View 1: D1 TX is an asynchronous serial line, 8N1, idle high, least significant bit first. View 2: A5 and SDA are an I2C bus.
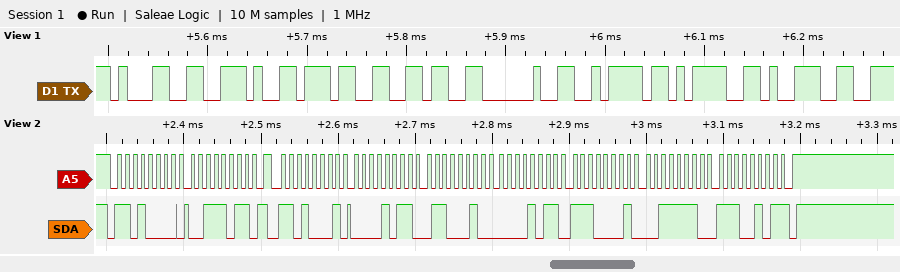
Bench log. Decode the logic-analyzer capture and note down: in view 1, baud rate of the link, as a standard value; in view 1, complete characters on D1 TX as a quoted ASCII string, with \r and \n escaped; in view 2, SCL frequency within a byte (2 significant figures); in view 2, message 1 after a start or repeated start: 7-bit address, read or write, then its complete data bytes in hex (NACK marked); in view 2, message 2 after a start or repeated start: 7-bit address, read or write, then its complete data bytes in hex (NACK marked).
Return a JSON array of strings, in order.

["115200 baud", "\"1.76 z=9\"", "100 kHz", "0x68 write: 3B", "0x68 read: 0B 62 0B E1 3E E5 NACK"]
